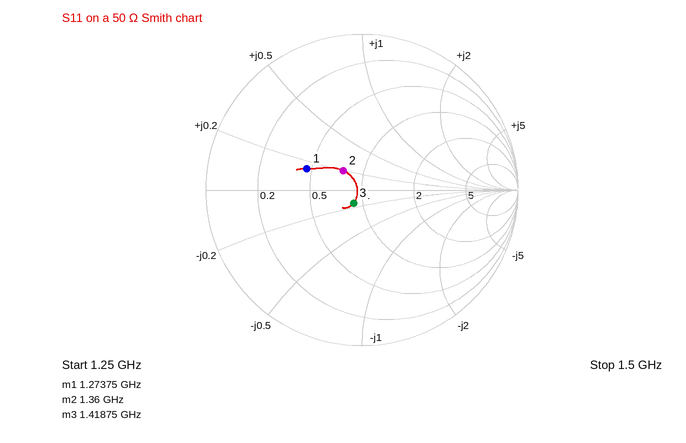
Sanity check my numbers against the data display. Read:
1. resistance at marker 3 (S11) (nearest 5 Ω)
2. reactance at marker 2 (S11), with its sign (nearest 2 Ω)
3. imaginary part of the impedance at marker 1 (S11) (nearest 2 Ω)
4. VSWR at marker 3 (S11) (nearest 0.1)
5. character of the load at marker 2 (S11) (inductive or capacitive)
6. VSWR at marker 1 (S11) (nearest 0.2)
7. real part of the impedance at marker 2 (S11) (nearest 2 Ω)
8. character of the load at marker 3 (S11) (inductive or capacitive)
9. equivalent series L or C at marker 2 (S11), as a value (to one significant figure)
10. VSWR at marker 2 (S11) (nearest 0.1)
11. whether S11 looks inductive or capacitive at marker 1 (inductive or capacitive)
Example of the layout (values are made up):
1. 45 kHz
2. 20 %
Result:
1. 45 Ω
2. +10 Ω
3. +8 Ω
4. 1.2
5. inductive
6. 2.2
7. 38 Ω
8. capacitive
9. 1 nH
10. 1.4
11. inductive
